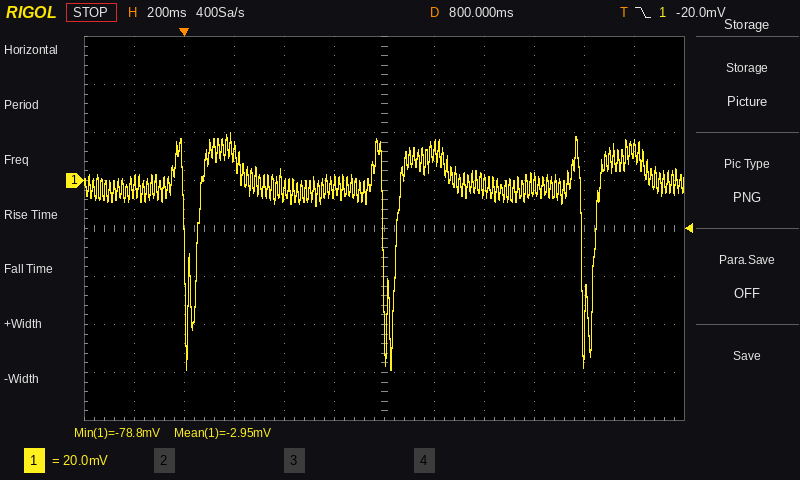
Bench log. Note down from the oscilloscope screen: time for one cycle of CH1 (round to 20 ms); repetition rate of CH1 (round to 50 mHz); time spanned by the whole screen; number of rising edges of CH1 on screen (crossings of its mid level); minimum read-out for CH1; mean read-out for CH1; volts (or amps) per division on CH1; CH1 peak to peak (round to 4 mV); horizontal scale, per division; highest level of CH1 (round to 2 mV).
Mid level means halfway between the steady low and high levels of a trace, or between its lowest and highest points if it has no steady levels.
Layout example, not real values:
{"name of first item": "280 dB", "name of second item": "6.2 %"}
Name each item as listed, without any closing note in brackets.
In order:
{"time for one cycle of CH1": "800 ms", "repetition rate of CH1": "1.25 Hz", "time spanned by the whole screen": "2.4 s", "number of rising edges of CH1 on screen": "3", "minimum read-out for CH1": "-78.8 mV", "mean read-out for CH1": "-2.95 mV", "volts (or amps) per division on CH1": "20 mV", "CH1 peak to peak": "100 mV", "horizontal scale, per division": "200 ms", "highest level of CH1": "20 mV"}
